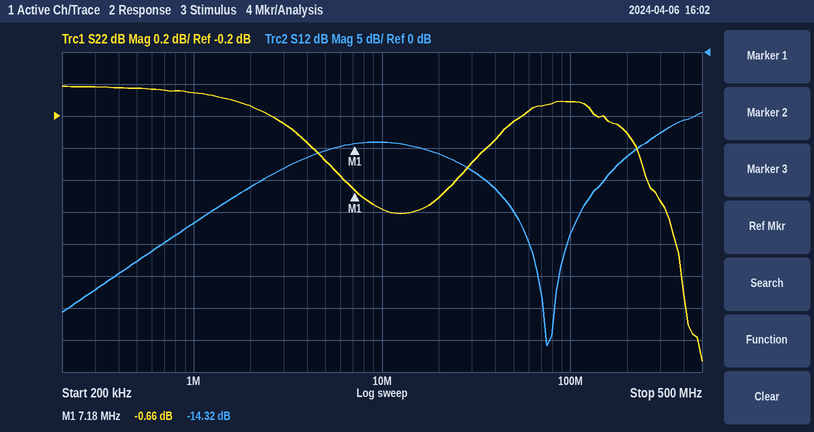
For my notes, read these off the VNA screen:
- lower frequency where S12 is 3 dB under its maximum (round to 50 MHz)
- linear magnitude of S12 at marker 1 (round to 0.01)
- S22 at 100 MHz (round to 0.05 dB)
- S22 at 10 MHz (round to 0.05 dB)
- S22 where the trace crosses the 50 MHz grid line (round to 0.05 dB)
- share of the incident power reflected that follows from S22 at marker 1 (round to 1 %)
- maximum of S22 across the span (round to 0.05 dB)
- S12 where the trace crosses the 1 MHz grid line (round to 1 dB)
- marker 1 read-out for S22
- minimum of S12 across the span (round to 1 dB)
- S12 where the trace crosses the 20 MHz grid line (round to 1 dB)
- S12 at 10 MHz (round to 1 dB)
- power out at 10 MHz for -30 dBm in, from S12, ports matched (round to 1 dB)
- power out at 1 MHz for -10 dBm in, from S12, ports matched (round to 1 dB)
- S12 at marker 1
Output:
300 MHz
0.19
-0.10 dB
-0.80 dB
-0.25 dB
86 %
0.00 dB
-27 dB
-0.66 dB
-46 dB
-16 dB
-14 dB
-44 dBm
-37 dBm
-14.32 dB
